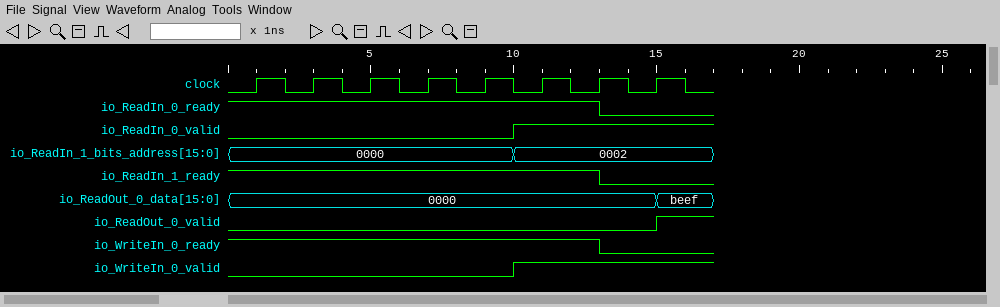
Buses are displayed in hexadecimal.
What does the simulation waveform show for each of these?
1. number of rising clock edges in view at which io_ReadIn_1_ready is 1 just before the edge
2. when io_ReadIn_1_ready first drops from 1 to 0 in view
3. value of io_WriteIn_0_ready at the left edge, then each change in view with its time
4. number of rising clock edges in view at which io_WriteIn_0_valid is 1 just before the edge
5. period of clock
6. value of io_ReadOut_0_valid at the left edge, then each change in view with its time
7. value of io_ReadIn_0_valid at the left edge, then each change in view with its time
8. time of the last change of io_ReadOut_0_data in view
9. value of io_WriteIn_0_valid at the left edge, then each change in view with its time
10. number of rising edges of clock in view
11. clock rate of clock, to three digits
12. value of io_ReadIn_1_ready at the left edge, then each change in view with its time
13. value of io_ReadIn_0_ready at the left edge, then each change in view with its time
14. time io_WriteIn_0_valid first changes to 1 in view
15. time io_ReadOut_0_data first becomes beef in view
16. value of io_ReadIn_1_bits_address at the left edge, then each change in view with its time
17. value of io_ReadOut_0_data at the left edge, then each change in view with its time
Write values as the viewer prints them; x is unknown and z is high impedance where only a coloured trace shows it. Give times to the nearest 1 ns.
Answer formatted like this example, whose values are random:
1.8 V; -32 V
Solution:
7; 13 ns; 1, 0 at 13 ns; 3; 2 ns; 0, 1 at 15 ns; 0, 1 at 10 ns; 15 ns; 0, 1 at 10 ns; 8; 500 MHz; 1, 0 at 13 ns; 1, 0 at 13 ns; 10 ns; 15 ns; 0000, 0002 at 10 ns; 0000, beef at 15 ns
